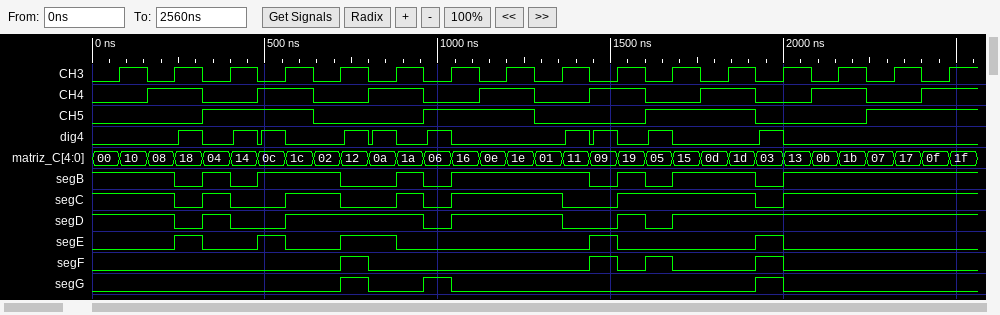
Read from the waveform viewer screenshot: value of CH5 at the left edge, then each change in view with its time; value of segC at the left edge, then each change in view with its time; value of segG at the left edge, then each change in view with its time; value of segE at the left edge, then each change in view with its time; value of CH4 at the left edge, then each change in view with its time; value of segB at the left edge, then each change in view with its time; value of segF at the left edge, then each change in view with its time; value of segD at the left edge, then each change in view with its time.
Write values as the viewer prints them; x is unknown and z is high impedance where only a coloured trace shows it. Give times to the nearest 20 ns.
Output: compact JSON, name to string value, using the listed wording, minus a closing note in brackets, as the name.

{"value of CH5 at the left edge, then each change in view with its time": "0, 1 at 320 ns, 0 at 640 ns, 1 at 960 ns, 0 at 1280 ns, 1 at 1600 ns, 0 at 1920 ns, 1 at 2240 ns", "value of segC at the left edge, then each change in view with its time": "1, 0 at 240 ns, 1 at 320 ns, 0 at 400 ns, 1 at 560 ns, 0 at 720 ns, 1 at 880 ns, 0 at 960 ns, 1 at 1040 ns, 0 at 1360 ns, 1 at 1520 ns, 0 at 1920 ns, 1 at 2000 ns", "value of segG at the left edge, then each change in view with its time": "0, 1 at 720 ns, 0 at 800 ns, 1 at 960 ns, 0 at 1040 ns, 1 at 1920 ns, 0 at 2000 ns", "value of segE at the left edge, then each change in view with its time": "0, 1 at 240 ns, 0 at 320 ns, 1 at 480 ns, 0 at 560 ns, 1 at 720 ns, 0 at 880 ns, 1 at 1440 ns, 0 at 1520 ns, 1 at 1920 ns, 0 at 2000 ns", "value of CH4 at the left edge, then each change in view with its time": "0, 1 at 160 ns, 0 at 320 ns, 1 at 480 ns, 0 at 640 ns, 1 at 800 ns, 0 at 960 ns, 1 at 1120 ns, 0 at 1280 ns, 1 at 1440 ns, 0 at 1600 ns, 1 at 1760 ns, 0 at 1920 ns, 1 at 2080 ns, 0 at 2240 ns, 1 at 2400 ns", "value of segB at the left edge, then each change in view with its time": "1, 0 at 240 ns, 1 at 320 ns, 0 at 400 ns, 1 at 480 ns, 0 at 720 ns, 1 at 880 ns, 0 at 960 ns, 1 at 1040 ns, 0 at 1440 ns, 1 at 1520 ns, 0 at 1600 ns, 1 at 1680 ns, 0 at 1920 ns, 1 at 2000 ns", "value of segF at the left edge, then each change in view with its time": "0, 1 at 720 ns, 0 at 800 ns, 1 at 1440 ns, 0 at 1520 ns, 1 at 1600 ns, 0 at 1680 ns, 1 at 1920 ns, 0 at 2000 ns", "value of segD at the left edge, then each change in view with its time": "1, 0 at 240 ns, 1 at 320 ns, 0 at 400 ns, 1 at 560 ns, 0 at 960 ns, 1 at 1040 ns, 0 at 1360 ns, 1 at 1520 ns, 0 at 1600 ns, 1 at 1680 ns"}
